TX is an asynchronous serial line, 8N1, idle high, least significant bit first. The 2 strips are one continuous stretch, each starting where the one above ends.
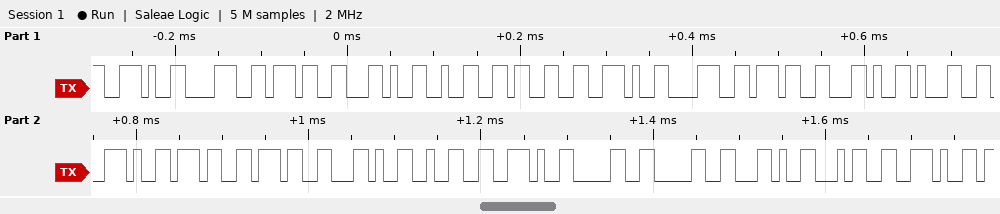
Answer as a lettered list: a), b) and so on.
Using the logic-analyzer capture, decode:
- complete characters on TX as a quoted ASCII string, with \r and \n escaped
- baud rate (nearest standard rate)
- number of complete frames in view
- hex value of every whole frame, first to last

a) ".87,23.87,1.77,2.00,4."
b) 115200 baud
c) 22
d) 0x2E 0x38 0x37 0x2C 0x32 0x33 0x2E 0x38 0x37 0x2C 0x31 0x2E 0x37 0x37 0x2C 0x32 0x2E 0x30 0x30 0x2C 0x34 0x2E
